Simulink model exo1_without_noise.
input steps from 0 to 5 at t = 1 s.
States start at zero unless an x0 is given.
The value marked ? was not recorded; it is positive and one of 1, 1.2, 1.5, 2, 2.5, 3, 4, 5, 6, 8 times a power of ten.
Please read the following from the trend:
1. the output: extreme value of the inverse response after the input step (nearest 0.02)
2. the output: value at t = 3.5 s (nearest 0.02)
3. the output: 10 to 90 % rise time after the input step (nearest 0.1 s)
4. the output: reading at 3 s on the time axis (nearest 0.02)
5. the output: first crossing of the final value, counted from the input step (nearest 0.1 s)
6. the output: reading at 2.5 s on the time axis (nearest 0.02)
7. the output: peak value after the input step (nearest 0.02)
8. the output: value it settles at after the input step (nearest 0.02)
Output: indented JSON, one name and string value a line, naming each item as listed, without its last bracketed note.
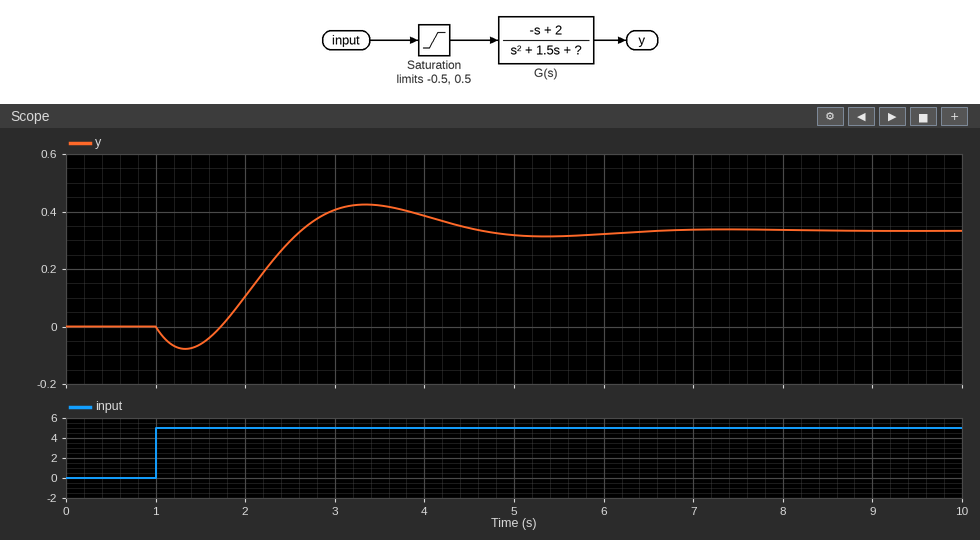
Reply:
{
  "the output: extreme value of the inverse response after the input step": "-0.08",
  "the output: value at t = 3.5 s": "0.42",
  "the output: 10 to 90 % rise time after the input step": "0.7 s",
  "the output: reading at 3 s on the time axis": "0.40",
  "the output: first crossing of the final value, counted from the input step": "1.6 s",
  "the output: reading at 2.5 s on the time axis": "0.30",
  "the output: peak value after the input step": "0.42",
  "the output: value it settles at after the input step": "0.34"
}
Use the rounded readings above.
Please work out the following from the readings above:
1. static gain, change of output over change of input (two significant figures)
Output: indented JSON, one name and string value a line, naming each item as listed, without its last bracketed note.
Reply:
{
  "static gain, change of output over change of input": "0.068"
}
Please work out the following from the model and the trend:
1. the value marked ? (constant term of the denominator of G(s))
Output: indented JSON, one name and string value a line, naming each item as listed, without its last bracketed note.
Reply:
{
  "the value marked ? (constant term of the denominator of G(s))": "3"
}
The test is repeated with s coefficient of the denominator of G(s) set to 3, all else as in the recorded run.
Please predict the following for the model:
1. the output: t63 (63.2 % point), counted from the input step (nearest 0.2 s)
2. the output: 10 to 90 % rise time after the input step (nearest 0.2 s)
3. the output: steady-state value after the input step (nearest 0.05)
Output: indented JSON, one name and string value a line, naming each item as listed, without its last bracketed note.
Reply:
{
  "the output: t63 (63.2 % point), counted from the input step": "1.6 s",
  "the output: 10 to 90 % rise time after the input step": "1.4 s",
  "the output: steady-state value after the input step": "0.35"
}
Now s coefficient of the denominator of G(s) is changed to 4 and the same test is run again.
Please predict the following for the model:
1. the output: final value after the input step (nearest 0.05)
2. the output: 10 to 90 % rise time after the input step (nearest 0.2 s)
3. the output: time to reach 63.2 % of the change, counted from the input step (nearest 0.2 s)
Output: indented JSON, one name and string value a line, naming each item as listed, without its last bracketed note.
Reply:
{
  "the output: final value after the input step": "0.35",
  "the output: 10 to 90 % rise time after the input step": "2.4 s",
  "the output: time to reach 63.2 % of the change, counted from the input step": "1.8 s"
}
